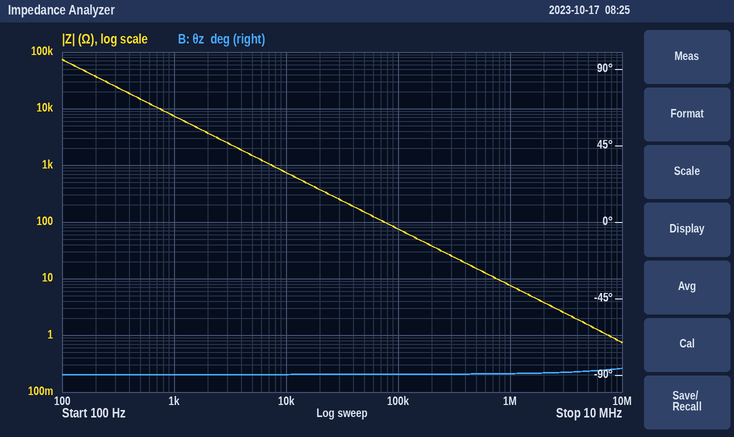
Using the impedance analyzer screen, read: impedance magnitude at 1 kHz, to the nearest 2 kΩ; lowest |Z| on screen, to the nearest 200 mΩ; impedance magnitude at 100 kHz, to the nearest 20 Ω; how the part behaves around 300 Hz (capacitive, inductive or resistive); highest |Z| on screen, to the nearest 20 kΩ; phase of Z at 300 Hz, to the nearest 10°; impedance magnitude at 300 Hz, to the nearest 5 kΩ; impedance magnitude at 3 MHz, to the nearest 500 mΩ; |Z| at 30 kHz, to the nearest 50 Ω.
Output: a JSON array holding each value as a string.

["8 kΩ", "800 mΩ", "80 Ω", "capacitive", "80 kΩ", "-90°", "25 kΩ", "2.5 Ω", "250 Ω"]
